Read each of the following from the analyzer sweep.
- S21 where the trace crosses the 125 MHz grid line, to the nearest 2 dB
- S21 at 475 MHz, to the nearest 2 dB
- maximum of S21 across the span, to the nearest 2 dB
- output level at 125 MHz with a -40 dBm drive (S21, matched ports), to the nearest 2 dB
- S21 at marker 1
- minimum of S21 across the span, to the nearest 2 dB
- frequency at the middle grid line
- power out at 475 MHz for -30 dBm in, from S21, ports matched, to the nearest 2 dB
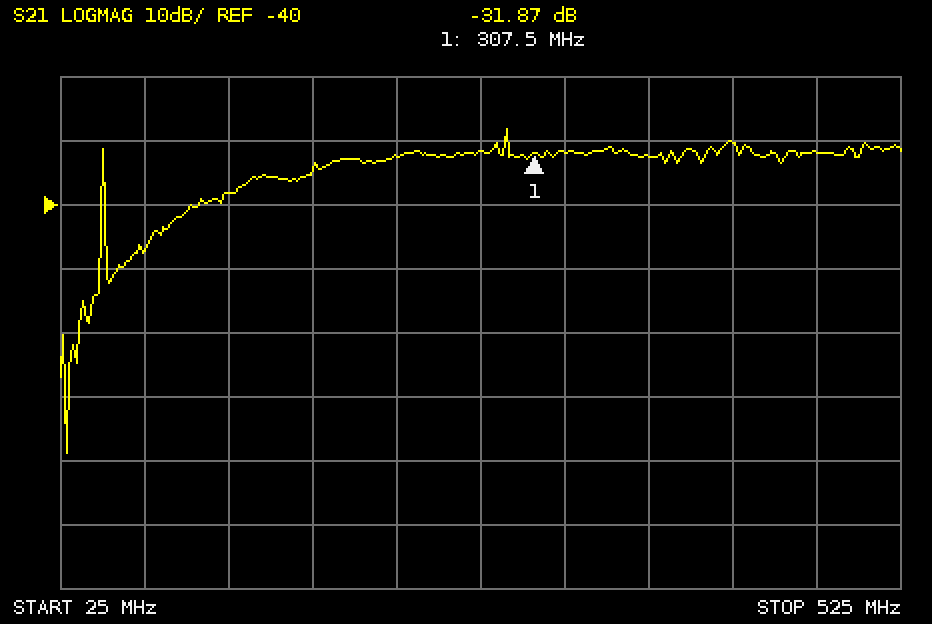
-38 dB
-32 dB
-28 dB
-78 dBm
-31.87 dB
-78 dB
275 MHz
-62 dBm
